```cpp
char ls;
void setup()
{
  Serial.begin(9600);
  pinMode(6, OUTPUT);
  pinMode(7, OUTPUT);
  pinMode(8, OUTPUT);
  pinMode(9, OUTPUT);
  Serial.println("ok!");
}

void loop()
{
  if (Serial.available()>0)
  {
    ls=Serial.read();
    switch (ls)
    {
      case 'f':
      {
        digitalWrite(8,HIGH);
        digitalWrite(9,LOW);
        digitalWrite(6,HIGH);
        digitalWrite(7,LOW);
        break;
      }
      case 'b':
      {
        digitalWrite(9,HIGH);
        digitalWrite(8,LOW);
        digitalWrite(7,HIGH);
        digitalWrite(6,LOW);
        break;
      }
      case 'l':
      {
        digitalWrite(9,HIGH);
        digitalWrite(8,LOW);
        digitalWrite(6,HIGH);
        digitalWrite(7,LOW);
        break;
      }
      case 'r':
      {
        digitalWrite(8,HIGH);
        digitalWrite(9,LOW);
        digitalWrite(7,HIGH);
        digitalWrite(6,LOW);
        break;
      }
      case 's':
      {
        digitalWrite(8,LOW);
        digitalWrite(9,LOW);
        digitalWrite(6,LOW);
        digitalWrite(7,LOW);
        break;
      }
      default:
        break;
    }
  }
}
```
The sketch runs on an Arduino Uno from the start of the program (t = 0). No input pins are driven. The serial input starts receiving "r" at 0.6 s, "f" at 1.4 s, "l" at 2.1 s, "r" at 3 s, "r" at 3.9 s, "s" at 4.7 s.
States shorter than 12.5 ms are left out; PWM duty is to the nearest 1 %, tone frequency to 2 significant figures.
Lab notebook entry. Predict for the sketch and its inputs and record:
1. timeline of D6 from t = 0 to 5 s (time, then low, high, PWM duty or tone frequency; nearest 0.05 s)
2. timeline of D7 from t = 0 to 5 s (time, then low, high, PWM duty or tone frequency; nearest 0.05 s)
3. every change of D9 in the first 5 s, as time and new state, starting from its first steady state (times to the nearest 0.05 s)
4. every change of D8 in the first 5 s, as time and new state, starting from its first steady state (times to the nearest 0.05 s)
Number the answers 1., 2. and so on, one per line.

1. 0 s low; 1.4 s high; 3 s low
2. 0 s low; 0.6 s high; 1.4 s low; 3 s high; 4.7 s low
3. 0 s low; 2.1 s high; 3 s low
4. 0 s low; 0.6 s high; 2.1 s low; 3 s high; 4.7 s low
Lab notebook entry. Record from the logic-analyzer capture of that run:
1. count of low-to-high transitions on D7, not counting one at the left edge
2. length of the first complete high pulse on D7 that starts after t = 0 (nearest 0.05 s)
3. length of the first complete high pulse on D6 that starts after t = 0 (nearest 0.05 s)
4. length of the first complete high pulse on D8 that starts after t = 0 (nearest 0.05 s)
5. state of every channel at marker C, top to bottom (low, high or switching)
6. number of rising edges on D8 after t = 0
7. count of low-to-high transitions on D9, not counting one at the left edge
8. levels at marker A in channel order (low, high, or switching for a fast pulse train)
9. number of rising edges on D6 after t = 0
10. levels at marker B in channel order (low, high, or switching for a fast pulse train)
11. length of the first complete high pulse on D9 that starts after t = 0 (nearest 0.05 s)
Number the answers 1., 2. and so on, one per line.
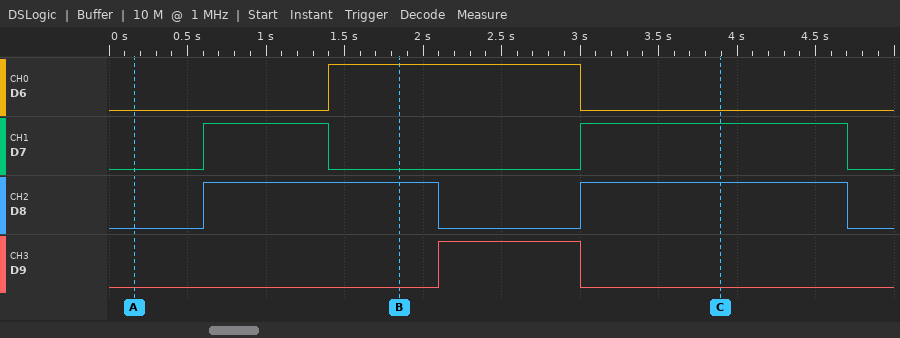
1. 2
2. 0.80 s
3. 1.60 s
4. 1.50 s
5. D6 low, D7 high, D8 high, D9 low
6. 2
7. 1
8. D6 low, D7 low, D8 low, D9 low
9. 1
10. D6 high, D7 low, D8 high, D9 low
11. 0.90 s
